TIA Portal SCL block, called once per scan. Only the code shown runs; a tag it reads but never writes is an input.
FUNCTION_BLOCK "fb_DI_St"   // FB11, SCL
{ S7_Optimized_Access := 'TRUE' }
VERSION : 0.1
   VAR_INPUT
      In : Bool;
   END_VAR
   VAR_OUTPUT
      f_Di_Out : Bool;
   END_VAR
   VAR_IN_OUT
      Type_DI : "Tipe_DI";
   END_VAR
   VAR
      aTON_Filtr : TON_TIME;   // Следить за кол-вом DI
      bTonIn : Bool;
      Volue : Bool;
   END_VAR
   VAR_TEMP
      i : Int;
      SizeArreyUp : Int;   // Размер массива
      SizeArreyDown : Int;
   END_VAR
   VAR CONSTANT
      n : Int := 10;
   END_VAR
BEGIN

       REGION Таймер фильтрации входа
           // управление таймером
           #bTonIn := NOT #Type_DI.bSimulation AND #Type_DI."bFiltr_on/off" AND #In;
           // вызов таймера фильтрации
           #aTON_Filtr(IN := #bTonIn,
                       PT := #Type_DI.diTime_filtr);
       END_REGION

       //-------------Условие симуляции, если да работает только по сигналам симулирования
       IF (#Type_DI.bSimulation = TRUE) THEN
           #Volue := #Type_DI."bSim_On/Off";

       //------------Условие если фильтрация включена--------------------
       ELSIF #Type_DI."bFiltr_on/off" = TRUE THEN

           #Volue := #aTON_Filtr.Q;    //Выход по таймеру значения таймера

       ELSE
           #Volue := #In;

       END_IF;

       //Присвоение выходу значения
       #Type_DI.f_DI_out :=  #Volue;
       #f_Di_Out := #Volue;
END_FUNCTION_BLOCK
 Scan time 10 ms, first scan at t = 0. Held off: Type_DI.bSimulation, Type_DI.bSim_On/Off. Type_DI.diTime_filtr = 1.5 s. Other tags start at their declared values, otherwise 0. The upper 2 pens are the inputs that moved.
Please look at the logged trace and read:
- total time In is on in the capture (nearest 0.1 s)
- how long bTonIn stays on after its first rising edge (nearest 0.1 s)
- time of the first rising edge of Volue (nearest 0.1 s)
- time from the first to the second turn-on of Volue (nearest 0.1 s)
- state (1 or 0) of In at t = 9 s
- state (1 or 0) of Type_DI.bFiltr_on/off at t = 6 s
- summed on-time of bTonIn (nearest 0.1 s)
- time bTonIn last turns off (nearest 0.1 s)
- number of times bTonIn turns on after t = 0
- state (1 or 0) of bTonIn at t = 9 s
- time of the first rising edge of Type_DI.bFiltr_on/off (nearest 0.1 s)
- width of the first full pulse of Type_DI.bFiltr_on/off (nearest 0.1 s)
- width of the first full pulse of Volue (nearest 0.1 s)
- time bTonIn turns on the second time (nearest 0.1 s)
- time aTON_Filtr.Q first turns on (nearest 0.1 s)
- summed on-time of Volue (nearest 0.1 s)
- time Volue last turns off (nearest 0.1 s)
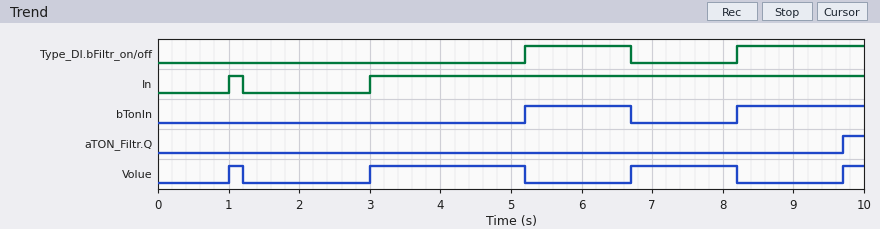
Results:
7.2 s
1.5 s
1.0 s
2.0 s
1
1
3.3 s
6.7 s
2
1
5.2 s
1.5 s
0.2 s
8.2 s
9.7 s
4.2 s
8.2 s
